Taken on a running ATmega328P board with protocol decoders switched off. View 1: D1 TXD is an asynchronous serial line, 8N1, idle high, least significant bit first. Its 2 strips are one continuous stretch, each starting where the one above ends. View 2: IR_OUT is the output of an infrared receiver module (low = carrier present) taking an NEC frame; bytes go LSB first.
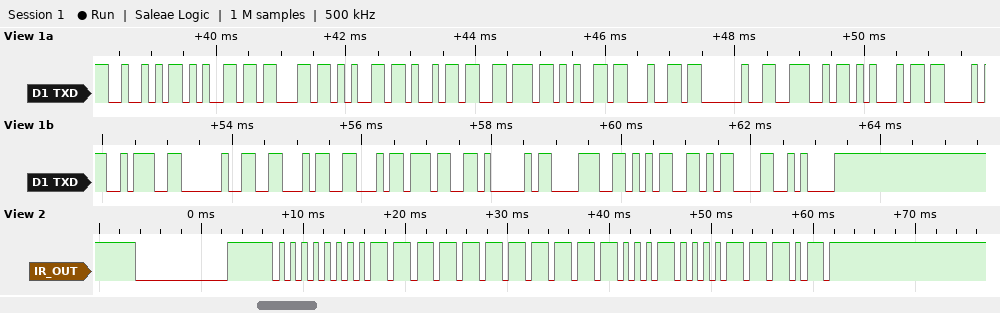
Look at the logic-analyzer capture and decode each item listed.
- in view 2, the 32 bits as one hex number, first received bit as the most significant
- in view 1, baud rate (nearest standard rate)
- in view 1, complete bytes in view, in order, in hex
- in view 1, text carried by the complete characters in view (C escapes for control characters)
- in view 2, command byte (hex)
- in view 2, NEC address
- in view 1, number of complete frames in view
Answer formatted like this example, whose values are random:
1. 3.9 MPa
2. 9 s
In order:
1. 0x00FFE21D
2. 9600 baud
3. 52 65 63 65 69 76 65 64 20 4E 45 43 3A 20 46 46 37 41 38 35 0D 0A
4. "Received NEC: FF7A85\r\n"
5. 0x47
6. 0x00
7. 22
